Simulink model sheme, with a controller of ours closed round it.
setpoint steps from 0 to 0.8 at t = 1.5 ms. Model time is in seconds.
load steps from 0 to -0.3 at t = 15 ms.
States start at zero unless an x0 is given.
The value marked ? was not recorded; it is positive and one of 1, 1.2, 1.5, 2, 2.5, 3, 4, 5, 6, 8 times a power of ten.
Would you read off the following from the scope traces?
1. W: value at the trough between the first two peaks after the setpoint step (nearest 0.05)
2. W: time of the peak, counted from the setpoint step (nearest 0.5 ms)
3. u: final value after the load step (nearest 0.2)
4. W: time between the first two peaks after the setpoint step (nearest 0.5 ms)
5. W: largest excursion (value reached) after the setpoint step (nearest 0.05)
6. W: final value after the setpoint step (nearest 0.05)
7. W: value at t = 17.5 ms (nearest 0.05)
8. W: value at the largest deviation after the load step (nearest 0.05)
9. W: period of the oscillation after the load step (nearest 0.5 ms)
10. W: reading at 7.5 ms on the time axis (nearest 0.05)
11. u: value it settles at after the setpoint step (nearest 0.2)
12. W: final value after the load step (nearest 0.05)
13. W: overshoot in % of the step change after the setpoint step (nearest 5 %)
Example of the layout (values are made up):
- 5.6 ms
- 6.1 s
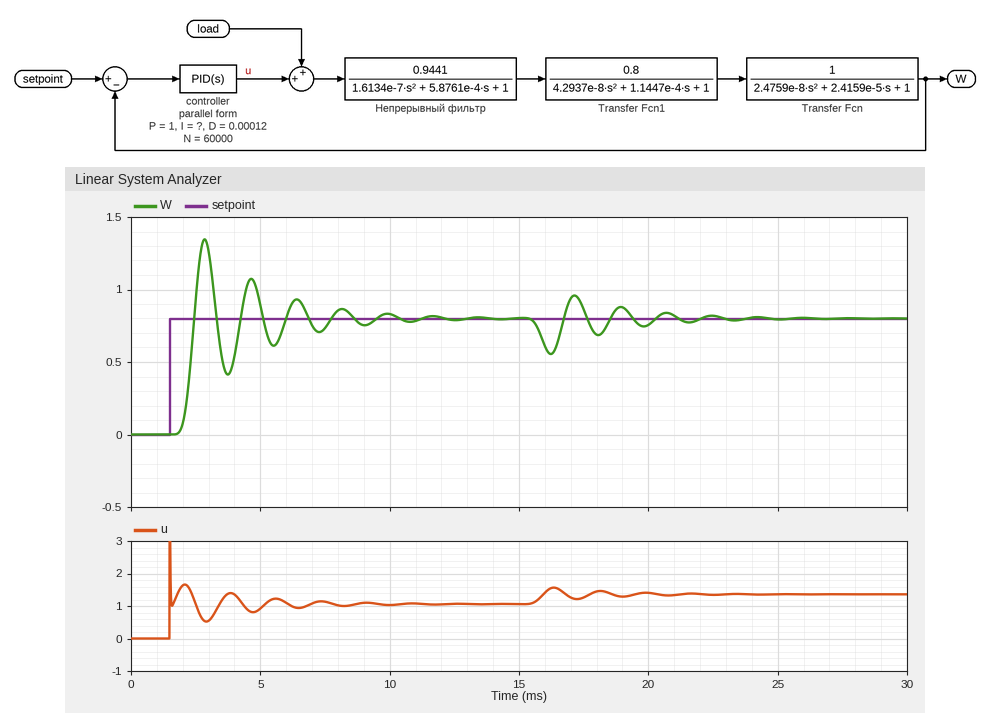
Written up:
- 0.40
- 1.5 ms
- 1.4
- 2.0 ms
- 1.35
- 0.80
- 0.85
- 0.55
- 2.0 ms
- 0.75
- 1.0
- 0.80
- 70 %
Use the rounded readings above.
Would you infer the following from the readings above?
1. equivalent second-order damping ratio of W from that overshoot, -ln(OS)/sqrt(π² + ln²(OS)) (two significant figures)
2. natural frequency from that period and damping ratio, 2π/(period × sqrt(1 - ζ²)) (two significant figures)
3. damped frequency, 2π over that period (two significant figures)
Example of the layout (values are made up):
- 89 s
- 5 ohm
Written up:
- 0.11
- 3.2 rad/ms
- 3.1 rad/ms
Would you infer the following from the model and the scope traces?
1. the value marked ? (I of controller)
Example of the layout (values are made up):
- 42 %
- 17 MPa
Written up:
- 2500
